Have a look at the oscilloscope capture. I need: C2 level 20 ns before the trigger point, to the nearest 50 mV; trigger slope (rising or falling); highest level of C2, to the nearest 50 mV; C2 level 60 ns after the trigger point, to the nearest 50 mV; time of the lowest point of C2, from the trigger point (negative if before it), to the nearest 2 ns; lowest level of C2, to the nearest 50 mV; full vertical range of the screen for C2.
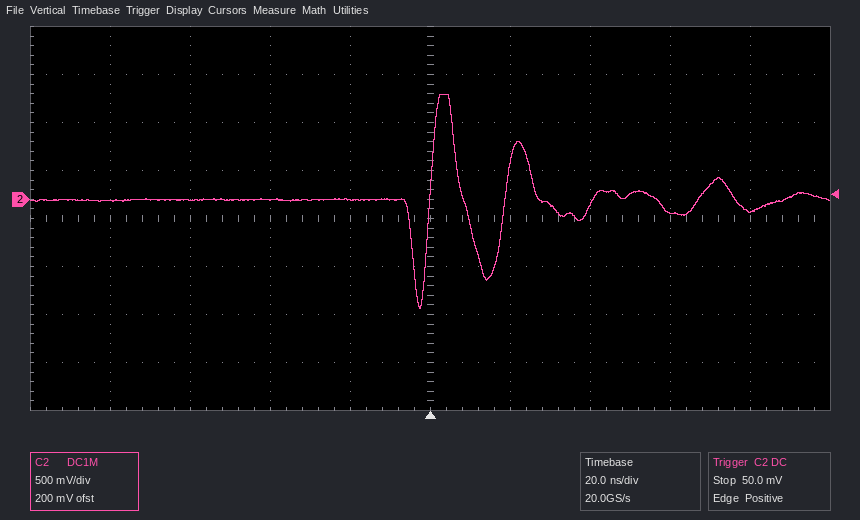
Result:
0 mV
rising
1.10 V
-150 mV
-2 ns
-1.15 V
4 V
